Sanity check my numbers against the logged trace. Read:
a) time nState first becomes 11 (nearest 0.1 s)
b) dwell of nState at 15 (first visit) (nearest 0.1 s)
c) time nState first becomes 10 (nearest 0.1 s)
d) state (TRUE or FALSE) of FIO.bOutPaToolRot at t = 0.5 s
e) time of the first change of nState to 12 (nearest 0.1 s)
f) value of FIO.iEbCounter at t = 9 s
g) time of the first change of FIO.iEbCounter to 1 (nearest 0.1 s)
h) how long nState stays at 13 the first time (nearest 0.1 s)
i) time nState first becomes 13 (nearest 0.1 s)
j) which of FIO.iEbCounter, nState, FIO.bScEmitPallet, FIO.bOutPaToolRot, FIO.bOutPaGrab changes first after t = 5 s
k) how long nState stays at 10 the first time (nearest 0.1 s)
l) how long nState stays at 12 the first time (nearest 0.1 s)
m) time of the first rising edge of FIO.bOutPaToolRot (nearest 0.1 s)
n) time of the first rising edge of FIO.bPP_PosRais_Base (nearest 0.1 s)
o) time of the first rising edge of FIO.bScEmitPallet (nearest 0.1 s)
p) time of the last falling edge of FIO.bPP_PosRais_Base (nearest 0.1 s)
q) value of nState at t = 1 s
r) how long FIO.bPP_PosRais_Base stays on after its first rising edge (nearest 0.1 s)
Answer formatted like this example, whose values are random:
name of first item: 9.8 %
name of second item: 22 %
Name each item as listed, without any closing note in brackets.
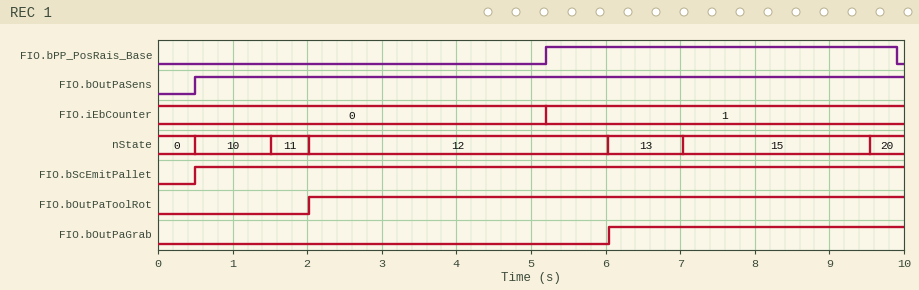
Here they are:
time nState first becomes 11: 1.5 s
dwell of nState at 15 (first visit): 2.5 s
time nState first becomes 10: 0.5 s
state (TRUE or FALSE) of FIO.bOutPaToolRot at t = 0.5 s: FALSE
time of the first change of nState to 12: 2.0 s
value of FIO.iEbCounter at t = 9 s: 1
time of the first change of FIO.iEbCounter to 1: 5.2 s
how long nState stays at 13 the first time: 1.0 s
time nState first becomes 13: 6.0 s
which of FIO.iEbCounter, nState, FIO.bScEmitPallet, FIO.bOutPaToolRot, FIO.bOutPaGrab changes first after t = 5 s: FIO.iEbCounter
how long nState stays at 10 the first time: 1.0 s
how long nState stays at 12 the first time: 4.0 s
time of the first rising edge of FIO.bOutPaToolRot: 2.0 s
time of the first rising edge of FIO.bPP_PosRais_Base: 5.2 s
time of the first rising edge of FIO.bScEmitPallet: 0.5 s
time of the last falling edge of FIO.bPP_PosRais_Base: 9.9 s
value of nState at t = 1 s: 10
how long FIO.bPP_PosRais_Base stays on after its first rising edge: 4.7 s
